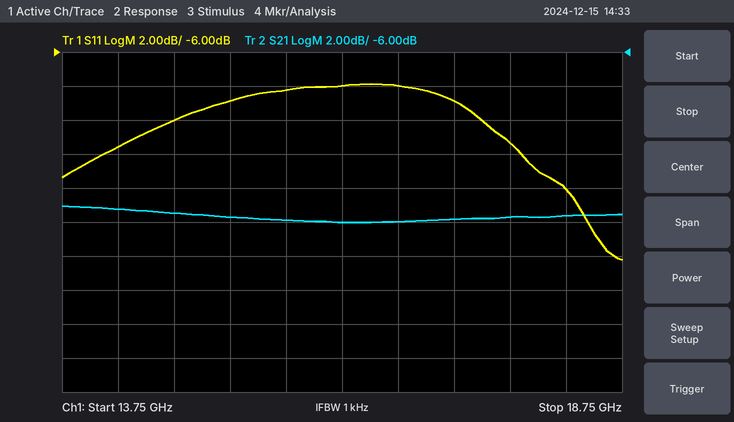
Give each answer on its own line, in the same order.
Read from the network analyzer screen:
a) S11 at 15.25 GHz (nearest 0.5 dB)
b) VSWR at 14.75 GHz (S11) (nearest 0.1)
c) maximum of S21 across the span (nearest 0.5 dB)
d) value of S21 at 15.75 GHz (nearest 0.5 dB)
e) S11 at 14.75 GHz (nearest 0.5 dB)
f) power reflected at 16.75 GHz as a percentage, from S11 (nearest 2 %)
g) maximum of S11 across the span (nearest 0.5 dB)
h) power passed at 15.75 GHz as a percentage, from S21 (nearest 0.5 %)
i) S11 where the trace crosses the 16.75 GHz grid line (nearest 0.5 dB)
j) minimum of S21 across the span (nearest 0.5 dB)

-9.0 dB
1.9
-15.0 dB
-16.0 dB
-10.0 dB
16 %
-8.0 dB
2.5 %
-8.0 dB
-16.0 dB
